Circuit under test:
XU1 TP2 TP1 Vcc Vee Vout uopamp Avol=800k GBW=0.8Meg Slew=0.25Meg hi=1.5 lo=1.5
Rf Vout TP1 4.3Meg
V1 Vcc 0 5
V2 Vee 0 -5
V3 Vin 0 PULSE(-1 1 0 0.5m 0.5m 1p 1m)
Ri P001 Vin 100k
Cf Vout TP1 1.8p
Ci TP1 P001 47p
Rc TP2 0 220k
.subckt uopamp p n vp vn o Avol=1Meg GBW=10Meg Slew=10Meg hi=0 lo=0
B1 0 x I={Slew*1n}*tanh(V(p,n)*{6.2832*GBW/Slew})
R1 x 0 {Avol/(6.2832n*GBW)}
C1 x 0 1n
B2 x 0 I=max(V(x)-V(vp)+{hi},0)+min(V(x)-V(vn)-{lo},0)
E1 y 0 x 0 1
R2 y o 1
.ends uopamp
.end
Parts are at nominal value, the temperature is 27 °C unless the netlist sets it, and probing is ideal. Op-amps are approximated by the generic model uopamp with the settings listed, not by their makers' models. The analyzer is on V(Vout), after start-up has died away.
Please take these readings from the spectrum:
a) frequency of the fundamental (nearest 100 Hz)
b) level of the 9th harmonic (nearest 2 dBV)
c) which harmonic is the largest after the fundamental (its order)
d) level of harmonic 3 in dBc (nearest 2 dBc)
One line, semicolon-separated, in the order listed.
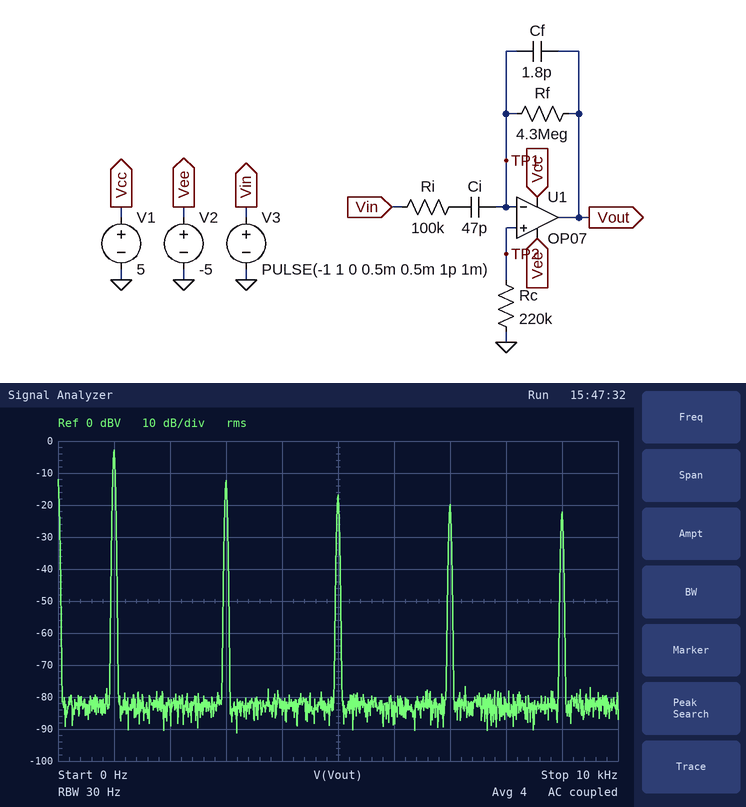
1.0 kHz; -22 dBV; 3; -10 dBc
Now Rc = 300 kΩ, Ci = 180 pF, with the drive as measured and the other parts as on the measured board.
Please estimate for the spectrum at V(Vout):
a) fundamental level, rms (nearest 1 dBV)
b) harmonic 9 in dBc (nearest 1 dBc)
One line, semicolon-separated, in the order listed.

9 dBV; -22 dBc
